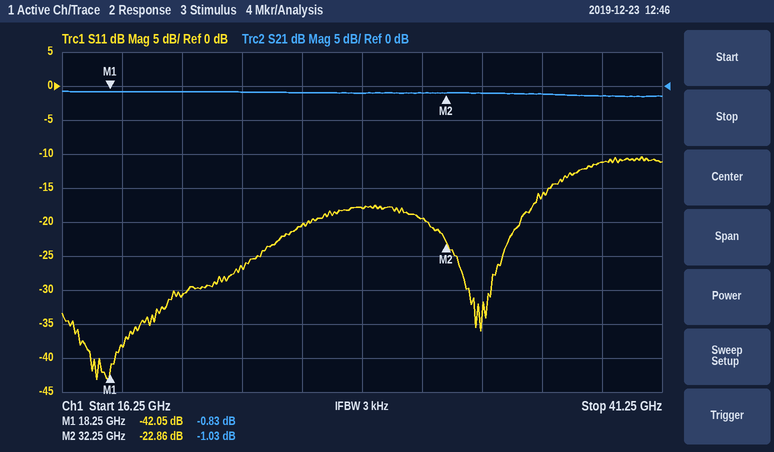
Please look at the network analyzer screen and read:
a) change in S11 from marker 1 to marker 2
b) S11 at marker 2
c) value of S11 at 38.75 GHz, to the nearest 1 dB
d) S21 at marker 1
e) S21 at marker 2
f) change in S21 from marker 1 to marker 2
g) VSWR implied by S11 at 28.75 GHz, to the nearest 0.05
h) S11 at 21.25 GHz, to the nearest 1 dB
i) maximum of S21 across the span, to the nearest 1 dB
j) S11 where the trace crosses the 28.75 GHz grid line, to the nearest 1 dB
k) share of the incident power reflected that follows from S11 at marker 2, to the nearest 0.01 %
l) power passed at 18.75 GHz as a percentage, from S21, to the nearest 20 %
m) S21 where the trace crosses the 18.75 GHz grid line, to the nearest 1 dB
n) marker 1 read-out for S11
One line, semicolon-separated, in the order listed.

19.19 dB; -22.86 dB; -11 dB; -0.83 dB; -1.03 dB; -0.20 dB; 1.30; -31 dB; -1 dB; -18 dB; 0.52 %; 80 %; -1 dB; -42.05 dB
